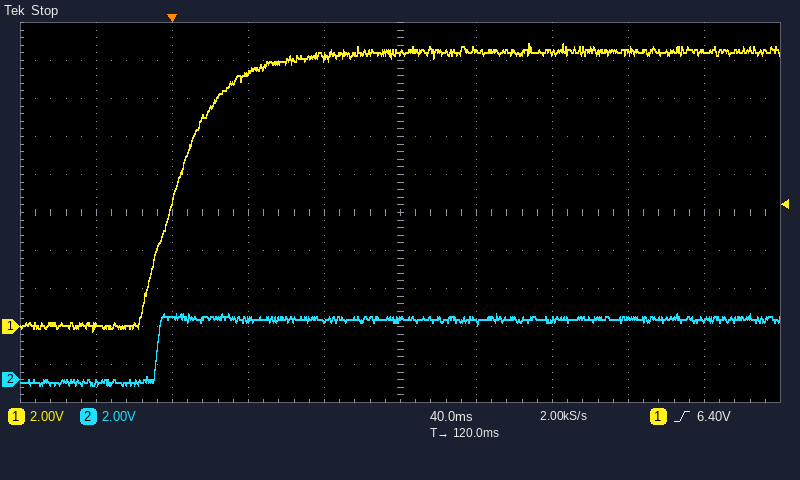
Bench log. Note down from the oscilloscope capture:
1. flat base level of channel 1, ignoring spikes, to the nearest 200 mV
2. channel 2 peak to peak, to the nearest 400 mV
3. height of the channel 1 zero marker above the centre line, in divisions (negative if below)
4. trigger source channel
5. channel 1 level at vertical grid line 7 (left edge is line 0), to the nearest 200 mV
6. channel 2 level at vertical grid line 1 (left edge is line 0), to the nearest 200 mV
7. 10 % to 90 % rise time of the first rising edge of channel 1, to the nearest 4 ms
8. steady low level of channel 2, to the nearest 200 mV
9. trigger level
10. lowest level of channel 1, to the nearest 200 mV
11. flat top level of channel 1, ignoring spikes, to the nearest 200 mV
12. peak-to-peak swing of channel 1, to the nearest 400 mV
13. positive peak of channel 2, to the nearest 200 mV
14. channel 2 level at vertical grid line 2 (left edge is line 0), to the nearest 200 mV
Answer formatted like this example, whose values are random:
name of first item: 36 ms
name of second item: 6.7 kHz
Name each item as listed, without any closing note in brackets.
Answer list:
flat base level of channel 1, ignoring spikes, to the nearest 200 mV: 0.0 V
channel 2 peak to peak, to the nearest 400 mV: 3.6 V
height of the channel 1 zero marker above the centre line, in divisions: -3.0 div
trigger source channel: channel 1
channel 1 level at vertical grid line 7 (left edge is line 0), to the nearest 200 mV: 14.4 V
channel 2 level at vertical grid line 1 (left edge is line 0), to the nearest 200 mV: -200 mV
10 % to 90 % rise time of the first rising edge of channel 1, to the nearest 4 ms: 48 ms
steady low level of channel 2, to the nearest 200 mV: -200 mV
trigger level: 6.40 V
lowest level of channel 1, to the nearest 200 mV: -200 mV
flat top level of channel 1, ignoring spikes, to the nearest 200 mV: 14.4 V
peak-to-peak swing of channel 1, to the nearest 400 mV: 15.2 V
positive peak of channel 2, to the nearest 200 mV: 3.4 V
channel 2 level at vertical grid line 2 (left edge is line 0), to the nearest 200 mV: 3.2 V
